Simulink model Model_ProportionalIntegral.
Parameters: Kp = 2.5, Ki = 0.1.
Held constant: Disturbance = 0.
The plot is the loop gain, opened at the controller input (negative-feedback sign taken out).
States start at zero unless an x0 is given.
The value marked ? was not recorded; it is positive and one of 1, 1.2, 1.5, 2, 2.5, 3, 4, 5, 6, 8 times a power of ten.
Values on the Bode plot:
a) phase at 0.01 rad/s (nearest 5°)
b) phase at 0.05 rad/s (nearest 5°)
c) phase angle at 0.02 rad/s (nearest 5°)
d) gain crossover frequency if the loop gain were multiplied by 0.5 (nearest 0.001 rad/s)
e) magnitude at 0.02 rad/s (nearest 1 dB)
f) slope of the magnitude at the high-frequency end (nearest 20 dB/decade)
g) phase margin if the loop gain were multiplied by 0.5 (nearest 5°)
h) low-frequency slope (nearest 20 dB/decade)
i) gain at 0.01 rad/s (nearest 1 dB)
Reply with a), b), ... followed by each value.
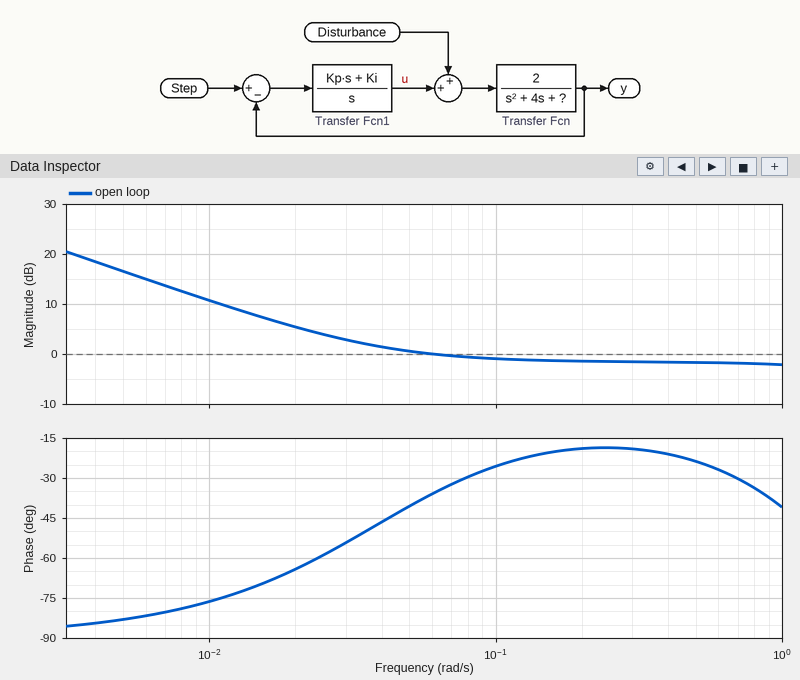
a) -75°
b) -40°
c) -65°
d) 0.018 rad/s
e) 5 dB
f) 0 dB/decade
g) 115°
h) -20 dB/decade
i) 11 dB
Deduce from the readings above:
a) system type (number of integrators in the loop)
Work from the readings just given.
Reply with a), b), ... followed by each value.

a) 1
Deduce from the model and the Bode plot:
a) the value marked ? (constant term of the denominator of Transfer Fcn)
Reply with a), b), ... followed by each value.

a) 6
